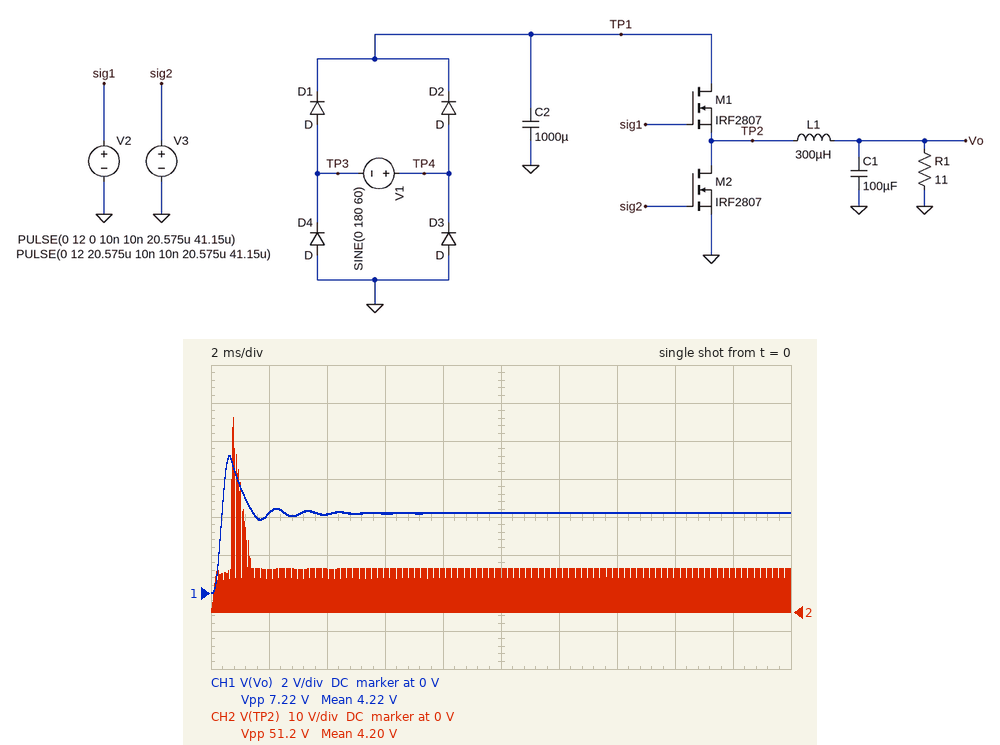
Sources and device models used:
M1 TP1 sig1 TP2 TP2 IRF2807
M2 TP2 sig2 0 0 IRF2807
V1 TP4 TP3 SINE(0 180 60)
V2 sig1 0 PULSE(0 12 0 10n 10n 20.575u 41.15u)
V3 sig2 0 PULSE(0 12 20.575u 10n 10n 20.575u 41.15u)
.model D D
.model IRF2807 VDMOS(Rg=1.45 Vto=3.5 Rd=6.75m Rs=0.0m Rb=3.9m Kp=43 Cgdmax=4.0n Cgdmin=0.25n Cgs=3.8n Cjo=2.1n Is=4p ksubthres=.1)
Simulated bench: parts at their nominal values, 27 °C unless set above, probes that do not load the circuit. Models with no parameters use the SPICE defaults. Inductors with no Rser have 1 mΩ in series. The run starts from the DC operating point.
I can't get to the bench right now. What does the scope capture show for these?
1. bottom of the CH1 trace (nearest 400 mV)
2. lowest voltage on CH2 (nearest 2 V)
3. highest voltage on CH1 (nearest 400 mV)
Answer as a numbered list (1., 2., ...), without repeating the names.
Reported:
1. 0 V
2. 0 V
3. 7.2 V
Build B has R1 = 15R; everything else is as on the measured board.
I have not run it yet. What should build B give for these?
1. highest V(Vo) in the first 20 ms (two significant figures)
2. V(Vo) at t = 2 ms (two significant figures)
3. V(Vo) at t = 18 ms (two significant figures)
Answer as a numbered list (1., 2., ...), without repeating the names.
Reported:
1. 7.4 V
2. 4.1 V
3. 4.2 V
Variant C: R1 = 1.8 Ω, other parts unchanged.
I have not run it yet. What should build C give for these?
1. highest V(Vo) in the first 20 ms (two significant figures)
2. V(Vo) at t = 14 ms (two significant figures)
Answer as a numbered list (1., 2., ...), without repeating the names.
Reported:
1. 4.8 V
2. 4.1 V
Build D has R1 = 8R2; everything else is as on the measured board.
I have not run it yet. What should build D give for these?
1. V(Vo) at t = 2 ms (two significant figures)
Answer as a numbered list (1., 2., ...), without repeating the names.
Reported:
1. 4.5 V
